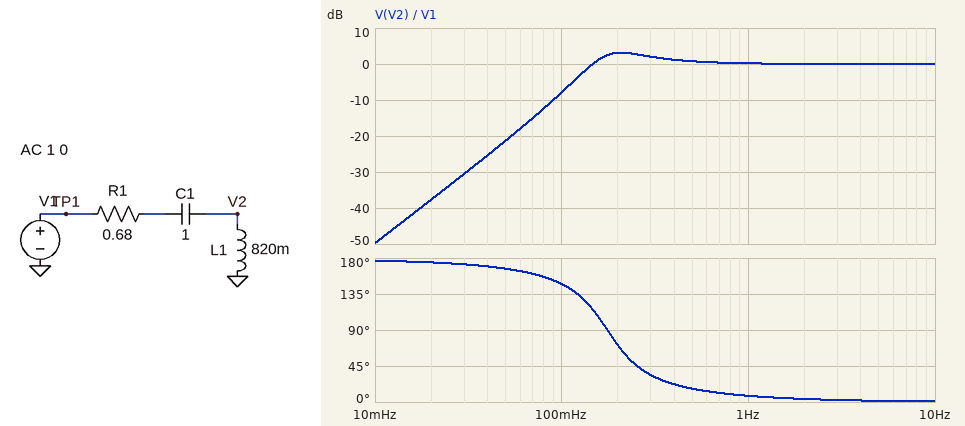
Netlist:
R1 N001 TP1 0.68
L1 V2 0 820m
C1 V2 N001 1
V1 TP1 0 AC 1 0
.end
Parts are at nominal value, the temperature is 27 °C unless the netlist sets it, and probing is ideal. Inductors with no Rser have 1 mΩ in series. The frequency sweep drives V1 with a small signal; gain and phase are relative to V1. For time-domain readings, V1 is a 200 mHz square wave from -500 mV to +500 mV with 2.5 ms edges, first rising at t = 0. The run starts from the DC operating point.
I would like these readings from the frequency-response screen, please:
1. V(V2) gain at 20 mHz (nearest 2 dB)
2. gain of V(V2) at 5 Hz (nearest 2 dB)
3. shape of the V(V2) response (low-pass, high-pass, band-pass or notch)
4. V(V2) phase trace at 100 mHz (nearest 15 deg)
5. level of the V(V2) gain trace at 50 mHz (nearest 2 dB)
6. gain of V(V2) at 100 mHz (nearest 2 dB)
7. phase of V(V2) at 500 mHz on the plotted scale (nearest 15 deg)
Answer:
-38 dB
0 dB
high-pass
150 deg
-22 dB
-8 dB
15 deg
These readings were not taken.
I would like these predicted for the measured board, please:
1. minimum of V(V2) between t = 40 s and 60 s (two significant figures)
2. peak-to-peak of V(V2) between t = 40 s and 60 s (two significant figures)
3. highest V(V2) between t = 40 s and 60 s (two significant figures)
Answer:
-1.5 V
2.9 V
1.5 V
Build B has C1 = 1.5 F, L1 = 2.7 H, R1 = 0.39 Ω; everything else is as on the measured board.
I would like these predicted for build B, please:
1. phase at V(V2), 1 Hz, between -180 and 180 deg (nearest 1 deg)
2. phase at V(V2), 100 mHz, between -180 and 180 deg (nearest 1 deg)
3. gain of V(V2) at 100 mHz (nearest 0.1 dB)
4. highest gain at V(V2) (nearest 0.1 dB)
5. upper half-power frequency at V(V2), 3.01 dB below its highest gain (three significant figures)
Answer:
1 deg
32 deg
7.1 dB
10.8 dB
96.7 mHz
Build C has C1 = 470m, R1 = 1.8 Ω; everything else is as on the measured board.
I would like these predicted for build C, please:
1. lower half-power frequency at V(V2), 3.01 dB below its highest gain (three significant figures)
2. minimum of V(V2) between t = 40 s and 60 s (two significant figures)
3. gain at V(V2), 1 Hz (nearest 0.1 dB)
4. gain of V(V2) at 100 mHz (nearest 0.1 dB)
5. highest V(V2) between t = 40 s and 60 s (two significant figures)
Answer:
248 mHz
-1.1 V
0 dB
-16.4 dB
1.1 V
